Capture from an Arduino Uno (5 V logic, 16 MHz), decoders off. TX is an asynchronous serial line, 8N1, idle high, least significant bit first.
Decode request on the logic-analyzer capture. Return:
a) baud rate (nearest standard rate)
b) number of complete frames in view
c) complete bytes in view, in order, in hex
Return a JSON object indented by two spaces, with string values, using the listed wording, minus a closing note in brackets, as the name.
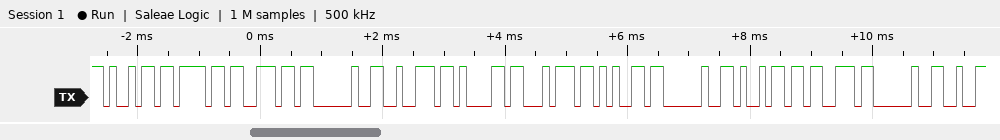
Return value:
{
  "baud rate": "9600 baud",
  "number of complete frames in view": "12",
  "complete bytes in view, in order, in hex": "0x69 0x6F 0x6E 0x20 0x72 0x61 0x74 0x65 0x20 0x69 0x73 0x20"
}
